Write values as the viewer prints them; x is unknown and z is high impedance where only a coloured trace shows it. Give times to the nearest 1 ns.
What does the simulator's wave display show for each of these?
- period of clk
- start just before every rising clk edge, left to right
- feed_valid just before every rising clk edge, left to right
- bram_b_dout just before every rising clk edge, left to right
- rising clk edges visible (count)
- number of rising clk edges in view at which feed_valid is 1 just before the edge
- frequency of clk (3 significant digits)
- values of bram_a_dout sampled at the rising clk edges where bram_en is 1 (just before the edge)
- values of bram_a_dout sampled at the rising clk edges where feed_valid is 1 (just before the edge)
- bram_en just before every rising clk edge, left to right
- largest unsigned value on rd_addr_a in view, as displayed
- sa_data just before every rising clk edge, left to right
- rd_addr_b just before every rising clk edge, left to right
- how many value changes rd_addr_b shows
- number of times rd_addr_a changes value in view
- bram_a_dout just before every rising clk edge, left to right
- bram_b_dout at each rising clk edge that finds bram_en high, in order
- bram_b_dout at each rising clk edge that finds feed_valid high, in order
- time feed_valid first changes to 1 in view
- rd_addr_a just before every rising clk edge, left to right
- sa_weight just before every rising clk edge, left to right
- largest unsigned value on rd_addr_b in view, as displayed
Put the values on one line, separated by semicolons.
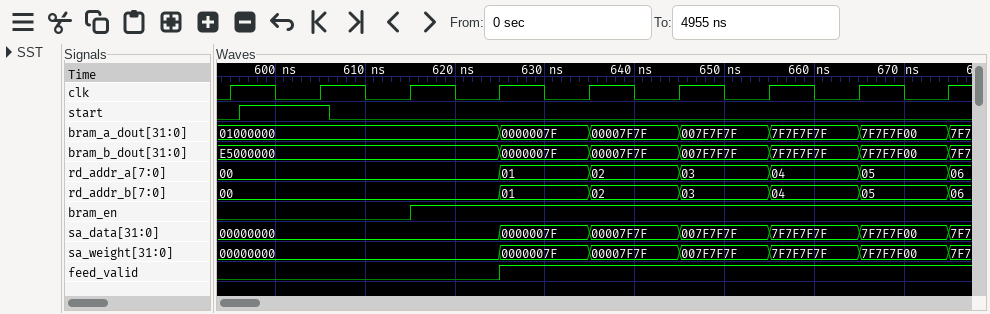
10 ns; 0 1 0 0 0 0 0 0 0; 0 0 0 0 1 1 1 1 1; E5000000, E5000000, E5000000, E5000000, 0000007F, 00007F7F, 007F7F7F, 7F7F7F7F, 7F7F7F00; 9; 5; 100 MHz; 01000000, 0000007F, 00007F7F, 007F7F7F, 7F7F7F7F, 7F7F7F00; 0000007F, 00007F7F, 007F7F7F, 7F7F7F7F, 7F7F7F00; 0 0 0 1 1 1 1 1 1; 06; 00000000, 00000000, 00000000, 00000000, 0000007F, 00007F7F, 007F7F7F, 7F7F7F7F, 7F7F7F00; 00, 00, 00, 00, 01, 02, 03, 04, 05; 6; 6; 01000000, 01000000, 01000000, 01000000, 0000007F, 00007F7F, 007F7F7F, 7F7F7F7F, 7F7F7F00; E5000000, 0000007F, 00007F7F, 007F7F7F, 7F7F7F7F, 7F7F7F00; 0000007F, 00007F7F, 007F7F7F, 7F7F7F7F, 7F7F7F00; 625 ns; 00, 00, 00, 00, 01, 02, 03, 04, 05; 00000000, 00000000, 00000000, 00000000, 0000007F, 00007F7F, 007F7F7F, 7F7F7F7F, 7F7F7F00; 06
